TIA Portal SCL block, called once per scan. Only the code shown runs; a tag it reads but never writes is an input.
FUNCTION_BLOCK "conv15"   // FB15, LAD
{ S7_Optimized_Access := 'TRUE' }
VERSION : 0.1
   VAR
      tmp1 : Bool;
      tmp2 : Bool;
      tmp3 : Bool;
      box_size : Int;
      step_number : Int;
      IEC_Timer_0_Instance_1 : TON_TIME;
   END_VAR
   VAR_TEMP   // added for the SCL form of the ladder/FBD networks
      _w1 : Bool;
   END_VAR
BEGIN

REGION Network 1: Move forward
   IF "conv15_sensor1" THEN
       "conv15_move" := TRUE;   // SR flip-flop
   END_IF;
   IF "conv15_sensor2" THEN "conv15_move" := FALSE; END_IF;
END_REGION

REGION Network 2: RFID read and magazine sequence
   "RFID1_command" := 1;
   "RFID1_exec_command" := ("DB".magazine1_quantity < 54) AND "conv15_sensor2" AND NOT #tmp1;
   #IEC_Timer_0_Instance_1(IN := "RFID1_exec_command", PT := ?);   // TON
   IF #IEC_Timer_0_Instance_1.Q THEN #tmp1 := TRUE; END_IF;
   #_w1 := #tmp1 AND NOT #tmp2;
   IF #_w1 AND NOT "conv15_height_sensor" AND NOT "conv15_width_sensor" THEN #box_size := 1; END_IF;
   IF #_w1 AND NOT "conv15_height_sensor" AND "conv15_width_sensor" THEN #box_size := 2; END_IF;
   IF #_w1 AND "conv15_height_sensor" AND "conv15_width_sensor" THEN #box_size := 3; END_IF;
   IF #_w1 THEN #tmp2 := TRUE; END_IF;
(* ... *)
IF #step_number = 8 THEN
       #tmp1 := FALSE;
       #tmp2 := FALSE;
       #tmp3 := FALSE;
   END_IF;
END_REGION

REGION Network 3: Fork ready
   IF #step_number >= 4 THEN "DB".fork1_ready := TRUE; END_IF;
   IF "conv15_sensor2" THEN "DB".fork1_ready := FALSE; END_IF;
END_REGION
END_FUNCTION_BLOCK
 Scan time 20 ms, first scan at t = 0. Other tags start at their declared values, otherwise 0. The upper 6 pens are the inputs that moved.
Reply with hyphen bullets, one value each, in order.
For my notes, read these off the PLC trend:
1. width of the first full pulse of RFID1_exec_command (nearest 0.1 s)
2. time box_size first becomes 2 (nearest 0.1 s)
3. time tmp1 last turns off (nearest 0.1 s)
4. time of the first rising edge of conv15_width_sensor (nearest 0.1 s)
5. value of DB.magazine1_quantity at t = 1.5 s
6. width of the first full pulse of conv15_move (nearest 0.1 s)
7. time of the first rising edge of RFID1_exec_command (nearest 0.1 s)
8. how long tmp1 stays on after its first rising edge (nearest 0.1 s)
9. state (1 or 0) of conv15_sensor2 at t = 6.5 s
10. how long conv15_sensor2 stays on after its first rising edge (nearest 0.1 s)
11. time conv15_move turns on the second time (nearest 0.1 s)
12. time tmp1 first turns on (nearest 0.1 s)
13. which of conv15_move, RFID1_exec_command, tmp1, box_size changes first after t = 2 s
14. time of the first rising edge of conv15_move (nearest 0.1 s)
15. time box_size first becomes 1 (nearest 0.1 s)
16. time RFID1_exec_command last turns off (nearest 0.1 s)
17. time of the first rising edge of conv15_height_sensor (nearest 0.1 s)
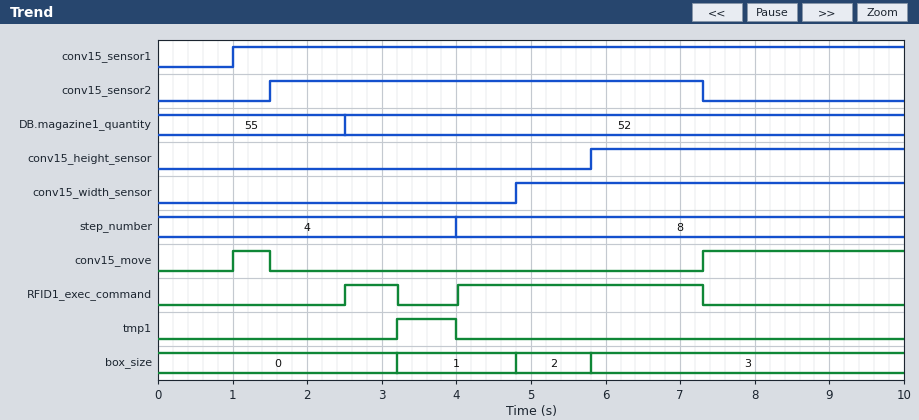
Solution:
- 0.7 s
- 4.8 s
- 4.0 s
- 4.8 s
- 55
- 0.5 s
- 2.5 s
- 0.8 s
- 1
- 5.8 s
- 7.3 s
- 3.2 s
- RFID1_exec_command
- 1.0 s
- 3.2 s
- 7.3 s
- 5.8 s
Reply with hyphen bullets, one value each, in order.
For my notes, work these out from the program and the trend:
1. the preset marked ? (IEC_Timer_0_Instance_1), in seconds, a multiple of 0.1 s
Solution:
- 0.7 s
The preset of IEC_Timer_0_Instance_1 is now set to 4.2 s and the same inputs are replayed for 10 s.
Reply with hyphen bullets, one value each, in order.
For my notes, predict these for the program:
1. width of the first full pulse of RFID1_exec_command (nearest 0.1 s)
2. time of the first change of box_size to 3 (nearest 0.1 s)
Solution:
- 4.8 s
- 6.7 s
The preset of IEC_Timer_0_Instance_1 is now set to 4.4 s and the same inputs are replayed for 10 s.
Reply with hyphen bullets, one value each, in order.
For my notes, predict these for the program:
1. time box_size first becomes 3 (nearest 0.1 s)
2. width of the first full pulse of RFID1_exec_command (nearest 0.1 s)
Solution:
- 6.9 s
- 4.8 s
